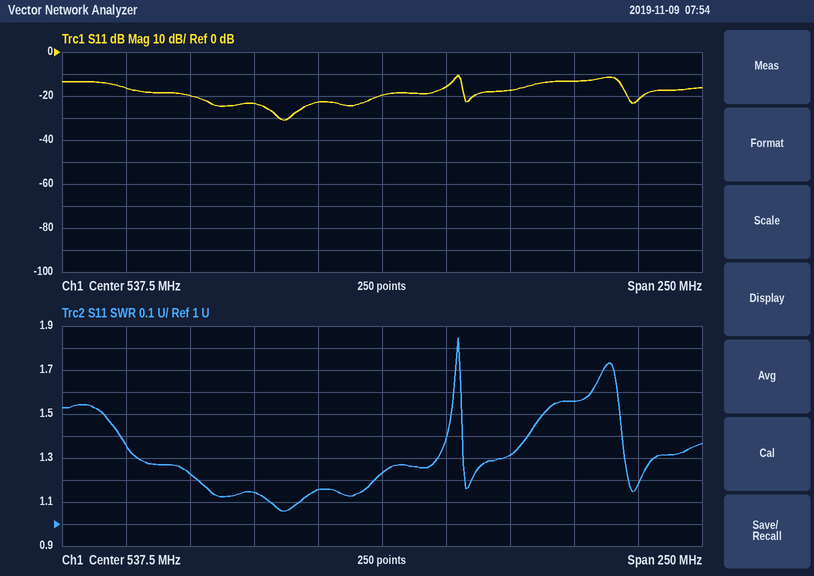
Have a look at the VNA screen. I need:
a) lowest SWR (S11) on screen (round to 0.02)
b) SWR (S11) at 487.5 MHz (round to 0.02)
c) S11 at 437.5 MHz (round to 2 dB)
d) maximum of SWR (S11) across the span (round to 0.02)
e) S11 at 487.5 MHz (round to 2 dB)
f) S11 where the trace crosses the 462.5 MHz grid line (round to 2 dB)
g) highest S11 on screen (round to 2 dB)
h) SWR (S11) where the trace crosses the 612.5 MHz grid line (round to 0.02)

1.06
1.14
-16 dB
1.84
-24 dB
-20 dB
-10 dB
1.56
